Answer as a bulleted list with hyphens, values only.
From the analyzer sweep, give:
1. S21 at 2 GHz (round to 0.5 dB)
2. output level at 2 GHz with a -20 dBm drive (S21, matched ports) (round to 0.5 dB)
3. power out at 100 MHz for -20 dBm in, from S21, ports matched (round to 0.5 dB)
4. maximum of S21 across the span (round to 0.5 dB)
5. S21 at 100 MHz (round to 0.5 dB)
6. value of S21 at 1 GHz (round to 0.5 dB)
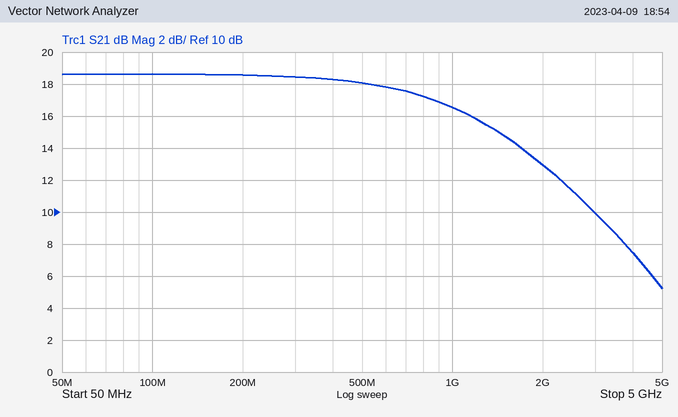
- 13.0 dB
- -7.0 dBm
- -1.5 dBm
- 18.5 dB
- 18.5 dB
- 16.5 dB
